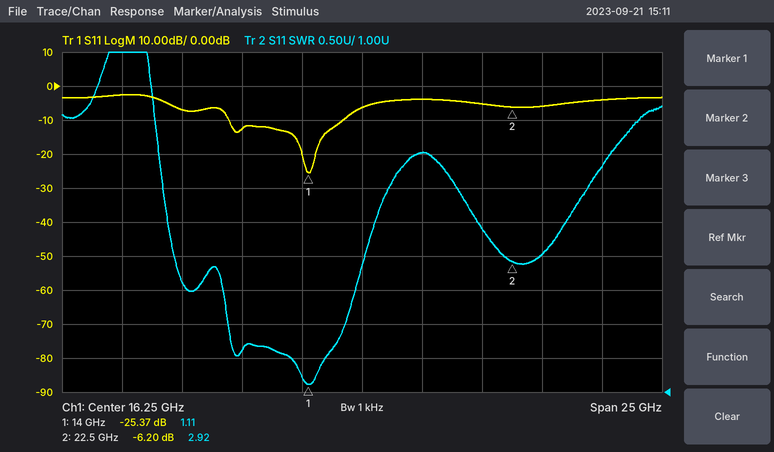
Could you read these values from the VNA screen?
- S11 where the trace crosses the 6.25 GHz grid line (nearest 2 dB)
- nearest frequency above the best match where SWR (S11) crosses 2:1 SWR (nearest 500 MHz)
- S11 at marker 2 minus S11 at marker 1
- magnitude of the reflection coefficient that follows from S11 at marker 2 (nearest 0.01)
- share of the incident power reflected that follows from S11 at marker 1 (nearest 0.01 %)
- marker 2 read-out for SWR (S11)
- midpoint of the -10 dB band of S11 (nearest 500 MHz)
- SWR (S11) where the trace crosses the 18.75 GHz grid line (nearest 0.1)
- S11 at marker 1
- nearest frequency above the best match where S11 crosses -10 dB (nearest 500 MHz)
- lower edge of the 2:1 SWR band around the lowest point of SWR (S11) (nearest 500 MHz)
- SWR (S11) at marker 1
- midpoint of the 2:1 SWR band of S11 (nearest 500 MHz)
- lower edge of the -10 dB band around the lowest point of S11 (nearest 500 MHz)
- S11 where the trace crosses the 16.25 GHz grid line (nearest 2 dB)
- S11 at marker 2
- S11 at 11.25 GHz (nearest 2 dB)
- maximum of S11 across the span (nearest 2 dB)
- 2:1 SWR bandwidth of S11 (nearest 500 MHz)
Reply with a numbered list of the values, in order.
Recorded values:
1. -2 dB
2. 15.5 GHz
3. 19.17 dB
4. 0.49
5. 0.29 %
6. 2.92
7. 13.0 GHz
8. 4.5
9. -25.37 dB
10. 15.5 GHz
11. 10.5 GHz
12. 1.11
13. 13.0 GHz
14. 10.5 GHz
15. -6 dB
16. -6.20 dB
17. -12 dB
18. -2 dB
19. 5.0 GHz
